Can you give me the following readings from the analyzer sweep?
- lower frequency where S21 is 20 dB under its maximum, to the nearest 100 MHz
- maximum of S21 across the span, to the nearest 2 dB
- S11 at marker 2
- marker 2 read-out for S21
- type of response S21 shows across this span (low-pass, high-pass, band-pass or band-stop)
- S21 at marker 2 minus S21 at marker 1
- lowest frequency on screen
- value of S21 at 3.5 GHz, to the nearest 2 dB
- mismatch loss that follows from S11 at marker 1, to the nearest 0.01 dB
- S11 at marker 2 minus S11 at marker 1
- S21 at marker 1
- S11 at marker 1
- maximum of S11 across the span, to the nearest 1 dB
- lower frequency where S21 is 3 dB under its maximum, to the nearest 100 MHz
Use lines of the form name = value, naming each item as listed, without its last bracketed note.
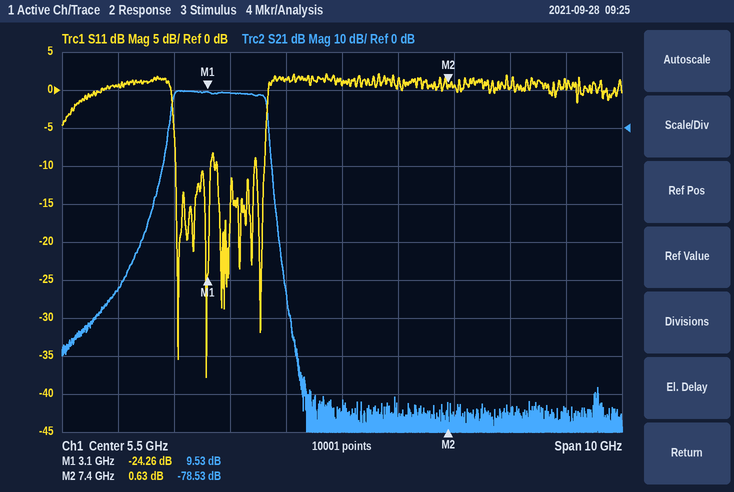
lower frequency where S21 is 20 dB under its maximum, to the nearest 100 MHz = 2.3 GHz
maximum of S21 across the span, to the nearest 2 dB = 10 dB
S11 at marker 2 = 0.63 dB
marker 2 read-out for S21 = -78.53 dB
type of response S21 shows across this span = band-pass
S21 at marker 2 minus S21 at marker 1 = -88.06 dB
lowest frequency on screen = 500 MHz
value of S21 at 3.5 GHz, to the nearest 2 dB = 10 dB
mismatch loss that follows from S11 at marker 1, to the nearest 0.01 dB = 0.02 dB
S11 at marker 2 minus S11 at marker 1 = 24.89 dB
S21 at marker 1 = 9.53 dB
S11 at marker 1 = -24.26 dB
maximum of S11 across the span, to the nearest 1 dB = 2 dB
lower frequency where S21 is 3 dB under its maximum, to the nearest 100 MHz = 2.5 GHz
